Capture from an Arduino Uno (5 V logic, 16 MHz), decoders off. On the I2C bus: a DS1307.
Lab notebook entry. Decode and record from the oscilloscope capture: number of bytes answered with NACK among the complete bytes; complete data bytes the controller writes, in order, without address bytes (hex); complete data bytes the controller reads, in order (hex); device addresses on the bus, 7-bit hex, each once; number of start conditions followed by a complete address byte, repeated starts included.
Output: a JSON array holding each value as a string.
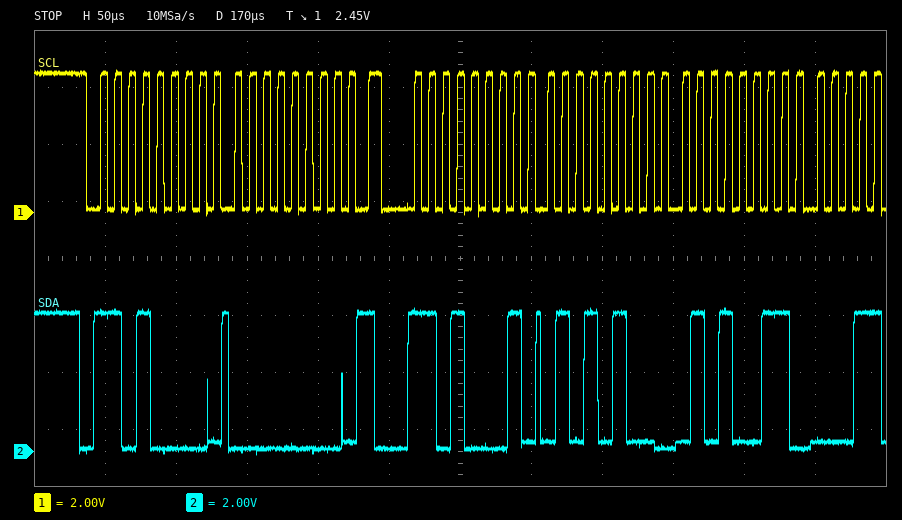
["0", "00", "54 53", "0x68", "2"]
